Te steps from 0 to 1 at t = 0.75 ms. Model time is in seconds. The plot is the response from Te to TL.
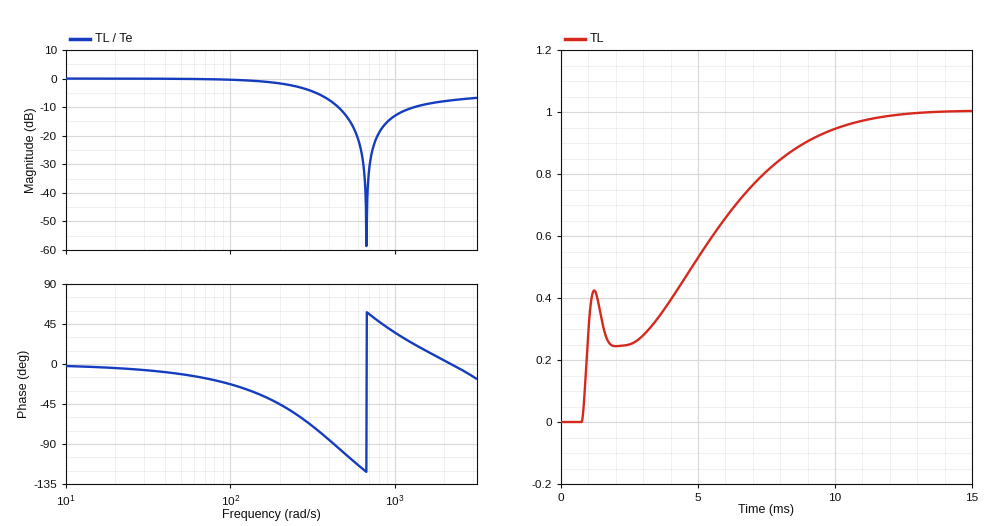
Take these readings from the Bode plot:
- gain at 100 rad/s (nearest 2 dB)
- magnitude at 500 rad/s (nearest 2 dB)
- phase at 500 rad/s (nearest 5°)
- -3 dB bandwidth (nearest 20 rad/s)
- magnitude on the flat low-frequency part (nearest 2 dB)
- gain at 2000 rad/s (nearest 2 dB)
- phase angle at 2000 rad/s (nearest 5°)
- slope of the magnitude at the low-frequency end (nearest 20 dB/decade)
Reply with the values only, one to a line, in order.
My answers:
0 dB
-12 dB
-100°
260 rad/s
0 dB
-8 dB
5°
0 dB/decade
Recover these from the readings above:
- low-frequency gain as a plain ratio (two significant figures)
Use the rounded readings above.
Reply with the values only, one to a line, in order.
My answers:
1.0
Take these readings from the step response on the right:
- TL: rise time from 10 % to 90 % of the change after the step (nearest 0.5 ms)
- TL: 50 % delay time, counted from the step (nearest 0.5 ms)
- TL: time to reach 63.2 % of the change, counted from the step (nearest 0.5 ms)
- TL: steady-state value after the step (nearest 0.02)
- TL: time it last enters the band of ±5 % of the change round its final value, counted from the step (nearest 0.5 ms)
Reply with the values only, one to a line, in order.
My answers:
8.0 ms
4.0 ms
5.0 ms
1.00
9.5 ms
